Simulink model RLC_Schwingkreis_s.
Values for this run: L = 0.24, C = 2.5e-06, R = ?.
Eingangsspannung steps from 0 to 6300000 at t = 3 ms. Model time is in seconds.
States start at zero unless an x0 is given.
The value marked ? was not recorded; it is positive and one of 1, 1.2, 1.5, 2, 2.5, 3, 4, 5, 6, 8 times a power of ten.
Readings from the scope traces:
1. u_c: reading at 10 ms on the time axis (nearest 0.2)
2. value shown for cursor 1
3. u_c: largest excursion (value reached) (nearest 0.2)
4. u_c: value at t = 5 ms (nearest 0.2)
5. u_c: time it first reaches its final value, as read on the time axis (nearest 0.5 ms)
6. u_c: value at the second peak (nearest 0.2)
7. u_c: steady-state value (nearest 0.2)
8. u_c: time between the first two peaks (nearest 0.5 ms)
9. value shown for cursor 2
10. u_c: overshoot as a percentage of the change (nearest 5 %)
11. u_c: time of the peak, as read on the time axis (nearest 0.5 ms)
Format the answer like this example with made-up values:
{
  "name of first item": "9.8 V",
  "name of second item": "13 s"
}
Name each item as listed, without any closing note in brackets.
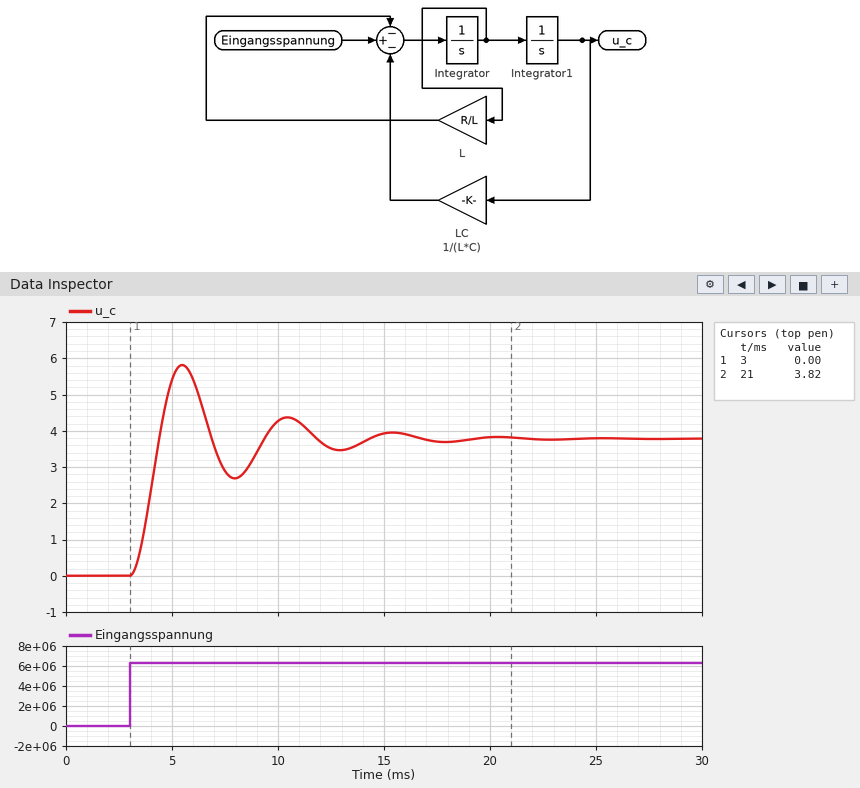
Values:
{
  "u_c: reading at 10 ms on the time axis": "4.2",
  "value shown for cursor 1": "0.00",
  "u_c: largest excursion (value reached)": "5.8",
  "u_c: value at t = 5 ms": "5.4",
  "u_c: time it first reaches its final value, as read on the time axis": "4.5 ms",
  "u_c: value at the second peak": "4.4",
  "u_c: steady-state value": "3.8",
  "u_c: time between the first two peaks": "5.0 ms",
  "value shown for cursor 2": "3.82",
  "u_c: overshoot as a percentage of the change": "55 %",
  "u_c: time of the peak, as read on the time axis": "5.5 ms"
}
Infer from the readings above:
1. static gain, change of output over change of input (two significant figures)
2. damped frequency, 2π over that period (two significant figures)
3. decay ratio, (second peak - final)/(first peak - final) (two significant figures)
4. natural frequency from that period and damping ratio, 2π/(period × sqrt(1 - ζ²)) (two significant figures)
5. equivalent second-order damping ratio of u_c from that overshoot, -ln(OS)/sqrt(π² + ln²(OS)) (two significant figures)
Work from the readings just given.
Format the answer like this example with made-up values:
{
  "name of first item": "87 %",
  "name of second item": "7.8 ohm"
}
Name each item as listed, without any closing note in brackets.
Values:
{
  "static gain, change of output over change of input": "0.00000060",
  "damped frequency, 2π over that period": "1.3 rad/ms",
  "decay ratio, (second peak - final)/(first peak - final)": "0.30",
  "natural frequency from that period and damping ratio, 2π/(period × sqrt(1 - ζ²))": "1.3 rad/ms",
  "equivalent second-order damping ratio of u_c from that overshoot, -ln(OS)/sqrt(π² + ln²(OS))": "0.19"
}
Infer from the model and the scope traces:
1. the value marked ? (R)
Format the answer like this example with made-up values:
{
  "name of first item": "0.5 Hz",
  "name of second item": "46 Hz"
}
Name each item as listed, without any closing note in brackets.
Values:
{
  "the value marked ?": "120"
}
